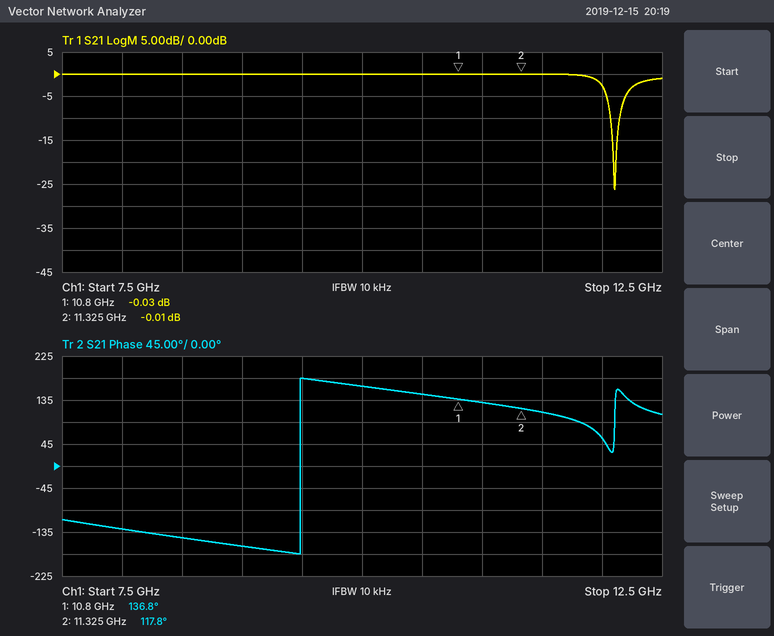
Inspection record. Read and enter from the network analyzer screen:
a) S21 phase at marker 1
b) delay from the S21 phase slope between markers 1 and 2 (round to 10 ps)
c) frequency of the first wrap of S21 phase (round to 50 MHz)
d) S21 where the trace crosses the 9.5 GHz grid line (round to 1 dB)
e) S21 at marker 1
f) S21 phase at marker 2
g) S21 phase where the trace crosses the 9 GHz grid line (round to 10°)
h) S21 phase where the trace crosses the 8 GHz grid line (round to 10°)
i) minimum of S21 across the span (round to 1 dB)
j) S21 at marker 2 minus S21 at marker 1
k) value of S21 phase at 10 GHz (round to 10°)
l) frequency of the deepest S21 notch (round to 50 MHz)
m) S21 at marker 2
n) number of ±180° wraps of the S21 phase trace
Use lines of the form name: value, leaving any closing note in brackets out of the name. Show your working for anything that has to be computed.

S21 phase at marker 1: 136.8°
delay from the S21 phase slope between markers 1 and 2: −(117.8° − (136.8°))/(360° × 525 MHz) ≈ 101 ps, so 100 ps to the nearest 10 ps
frequency of the first wrap of S21 phase: 9.50 GHz
S21 where the trace crosses the 9.5 GHz grid line: 0 dB
S21 at marker 1: -0.03 dB
S21 phase at marker 2: 117.8°
S21 phase where the trace crosses the 9 GHz grid line: -160°
S21 phase where the trace crosses the 8 GHz grid line: -130°
minimum of S21 across the span: -26 dB
S21 at marker 2 minus S21 at marker 1: -0.01 − (-0.03) = 0.02 dB
value of S21 phase at 10 GHz: 160°
frequency of the deepest S21 notch: 12.10 GHz
S21 at marker 2: -0.01 dB
number of ±180° wraps of the S21 phase trace: 1
